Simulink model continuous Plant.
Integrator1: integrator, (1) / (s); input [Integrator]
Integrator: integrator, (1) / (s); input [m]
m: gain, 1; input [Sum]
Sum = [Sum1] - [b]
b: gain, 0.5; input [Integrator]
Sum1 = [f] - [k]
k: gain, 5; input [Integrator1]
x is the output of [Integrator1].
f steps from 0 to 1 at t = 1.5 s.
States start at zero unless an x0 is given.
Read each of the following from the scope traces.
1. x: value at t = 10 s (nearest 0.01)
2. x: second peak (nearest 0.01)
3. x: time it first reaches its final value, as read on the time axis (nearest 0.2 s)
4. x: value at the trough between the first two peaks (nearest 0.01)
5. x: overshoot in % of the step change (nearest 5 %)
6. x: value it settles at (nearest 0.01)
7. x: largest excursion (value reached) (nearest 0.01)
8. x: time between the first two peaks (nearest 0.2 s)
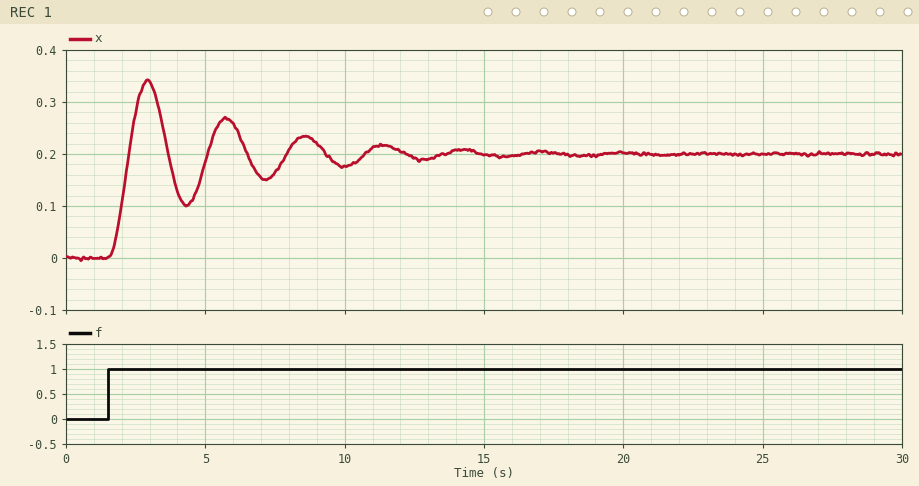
0.18
0.27
2.2 s
0.10
70 %
0.20
0.34
2.8 s
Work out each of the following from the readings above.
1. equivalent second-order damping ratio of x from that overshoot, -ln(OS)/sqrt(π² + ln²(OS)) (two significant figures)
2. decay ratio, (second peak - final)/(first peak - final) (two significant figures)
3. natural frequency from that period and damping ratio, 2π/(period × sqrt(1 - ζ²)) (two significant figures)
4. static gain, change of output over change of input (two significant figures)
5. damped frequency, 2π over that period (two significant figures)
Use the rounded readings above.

0.11
0.50
2.3 rad/s
0.20
2.2 rad/s
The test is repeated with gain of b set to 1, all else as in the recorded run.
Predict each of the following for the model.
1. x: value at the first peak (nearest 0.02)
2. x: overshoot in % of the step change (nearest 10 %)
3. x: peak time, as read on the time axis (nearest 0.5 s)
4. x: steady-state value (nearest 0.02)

0.30
50 %
3.0 s
0.20
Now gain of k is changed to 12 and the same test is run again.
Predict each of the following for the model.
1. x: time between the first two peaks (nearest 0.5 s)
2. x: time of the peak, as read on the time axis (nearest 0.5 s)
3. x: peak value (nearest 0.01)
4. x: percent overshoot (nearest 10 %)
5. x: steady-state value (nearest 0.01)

2.0 s
2.5 s
0.15
80 %
0.08
